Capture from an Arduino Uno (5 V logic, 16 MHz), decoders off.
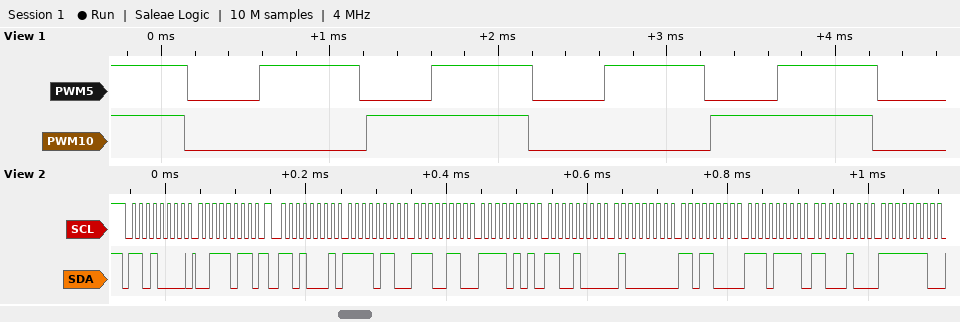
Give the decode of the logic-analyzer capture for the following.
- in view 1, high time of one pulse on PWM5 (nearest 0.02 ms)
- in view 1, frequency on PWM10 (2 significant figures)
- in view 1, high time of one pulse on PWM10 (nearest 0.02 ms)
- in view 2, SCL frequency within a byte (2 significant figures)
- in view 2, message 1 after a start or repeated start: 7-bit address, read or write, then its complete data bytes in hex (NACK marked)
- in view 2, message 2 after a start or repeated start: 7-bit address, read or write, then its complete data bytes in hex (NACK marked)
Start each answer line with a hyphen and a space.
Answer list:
- 0.60 ms
- 490 Hz
- 0.96 ms
- 100 kHz
- 0x68 write: 3B
- 0x68 read: F6 E6 F5 C8 40 D8 EF C4 FE
